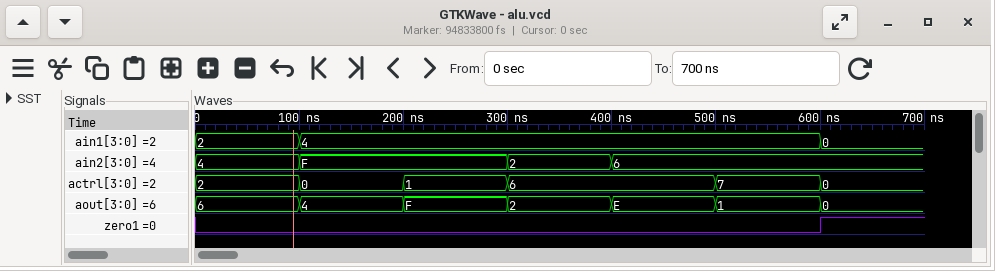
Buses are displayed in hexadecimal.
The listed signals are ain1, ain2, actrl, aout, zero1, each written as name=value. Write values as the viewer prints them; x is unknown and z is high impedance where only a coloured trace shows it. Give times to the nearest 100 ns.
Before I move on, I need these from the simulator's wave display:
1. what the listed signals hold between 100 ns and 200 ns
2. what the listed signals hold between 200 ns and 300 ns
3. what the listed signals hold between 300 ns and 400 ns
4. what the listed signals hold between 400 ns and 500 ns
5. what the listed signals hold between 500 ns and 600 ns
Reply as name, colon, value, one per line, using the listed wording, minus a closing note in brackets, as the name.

what the listed signals hold between 100 ns and 200 ns: ain1=4, ain2=F, actrl=0, aout=4, zero1=0
what the listed signals hold between 200 ns and 300 ns: ain1=4, ain2=F, actrl=1, aout=F, zero1=0
what the listed signals hold between 300 ns and 400 ns: ain1=4, ain2=2, actrl=6, aout=2, zero1=0
what the listed signals hold between 400 ns and 500 ns: ain1=4, ain2=6, actrl=6, aout=E, zero1=0
what the listed signals hold between 500 ns and 600 ns: ain1=4, ain2=6, actrl=7, aout=1, zero1=0
